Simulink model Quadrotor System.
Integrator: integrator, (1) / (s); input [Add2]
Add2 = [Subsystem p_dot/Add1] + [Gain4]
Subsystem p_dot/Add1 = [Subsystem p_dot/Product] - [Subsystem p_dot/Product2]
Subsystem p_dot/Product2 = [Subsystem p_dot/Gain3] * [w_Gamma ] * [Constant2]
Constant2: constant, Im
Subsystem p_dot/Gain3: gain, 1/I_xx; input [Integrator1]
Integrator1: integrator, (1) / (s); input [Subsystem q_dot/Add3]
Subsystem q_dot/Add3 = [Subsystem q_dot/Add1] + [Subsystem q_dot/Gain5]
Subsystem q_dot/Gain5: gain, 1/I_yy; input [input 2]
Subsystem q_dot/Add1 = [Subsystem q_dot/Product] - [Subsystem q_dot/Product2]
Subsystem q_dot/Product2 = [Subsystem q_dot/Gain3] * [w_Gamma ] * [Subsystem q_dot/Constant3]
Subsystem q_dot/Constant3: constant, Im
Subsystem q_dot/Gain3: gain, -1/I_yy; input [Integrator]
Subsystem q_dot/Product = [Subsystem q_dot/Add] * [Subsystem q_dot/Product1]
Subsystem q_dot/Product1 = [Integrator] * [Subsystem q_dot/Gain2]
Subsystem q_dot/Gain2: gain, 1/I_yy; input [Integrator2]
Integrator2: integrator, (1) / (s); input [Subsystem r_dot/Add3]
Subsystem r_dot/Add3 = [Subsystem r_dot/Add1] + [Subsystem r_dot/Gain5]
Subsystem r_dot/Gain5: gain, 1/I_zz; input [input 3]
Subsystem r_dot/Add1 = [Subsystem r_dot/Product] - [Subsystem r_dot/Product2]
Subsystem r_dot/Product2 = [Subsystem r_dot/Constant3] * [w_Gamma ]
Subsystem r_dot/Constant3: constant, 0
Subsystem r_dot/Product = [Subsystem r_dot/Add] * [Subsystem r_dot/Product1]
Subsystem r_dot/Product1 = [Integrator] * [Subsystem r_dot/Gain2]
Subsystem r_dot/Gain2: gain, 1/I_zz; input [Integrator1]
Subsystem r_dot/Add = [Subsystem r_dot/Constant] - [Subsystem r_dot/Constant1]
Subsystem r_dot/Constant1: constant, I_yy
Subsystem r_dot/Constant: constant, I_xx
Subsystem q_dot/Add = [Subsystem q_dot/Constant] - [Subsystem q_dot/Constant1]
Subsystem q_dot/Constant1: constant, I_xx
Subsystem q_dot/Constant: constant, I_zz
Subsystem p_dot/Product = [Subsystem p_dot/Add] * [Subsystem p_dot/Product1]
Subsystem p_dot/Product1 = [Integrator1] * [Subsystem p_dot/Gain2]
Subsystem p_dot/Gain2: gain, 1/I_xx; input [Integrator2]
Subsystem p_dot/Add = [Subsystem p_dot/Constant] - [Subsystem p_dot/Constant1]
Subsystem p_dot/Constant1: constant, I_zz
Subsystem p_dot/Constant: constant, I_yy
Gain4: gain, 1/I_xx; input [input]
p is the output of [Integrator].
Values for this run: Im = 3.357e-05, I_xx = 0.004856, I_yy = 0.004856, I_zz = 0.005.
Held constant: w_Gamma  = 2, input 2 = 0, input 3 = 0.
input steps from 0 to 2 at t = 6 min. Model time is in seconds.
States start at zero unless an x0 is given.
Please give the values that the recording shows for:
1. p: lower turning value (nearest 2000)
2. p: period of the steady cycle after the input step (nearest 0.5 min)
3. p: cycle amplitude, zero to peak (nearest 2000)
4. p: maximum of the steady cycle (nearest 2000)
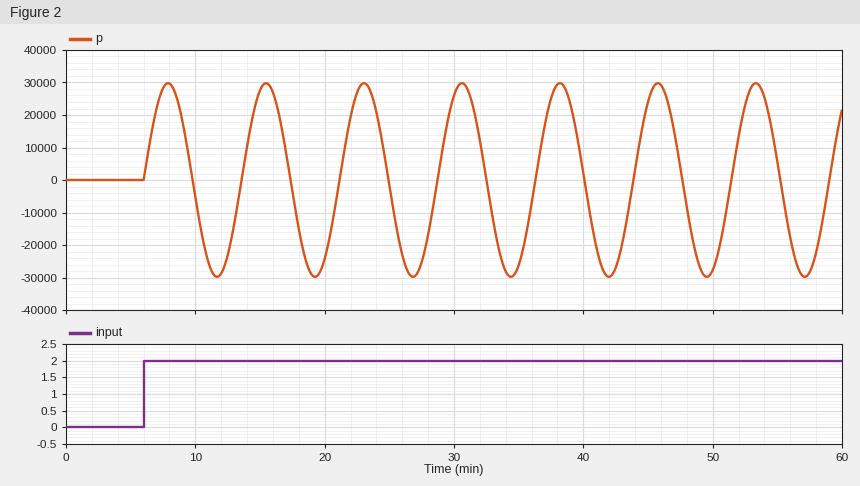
-30000
7.5 min
30000
30000
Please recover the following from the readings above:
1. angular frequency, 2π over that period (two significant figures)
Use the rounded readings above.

0.84 rad/min
